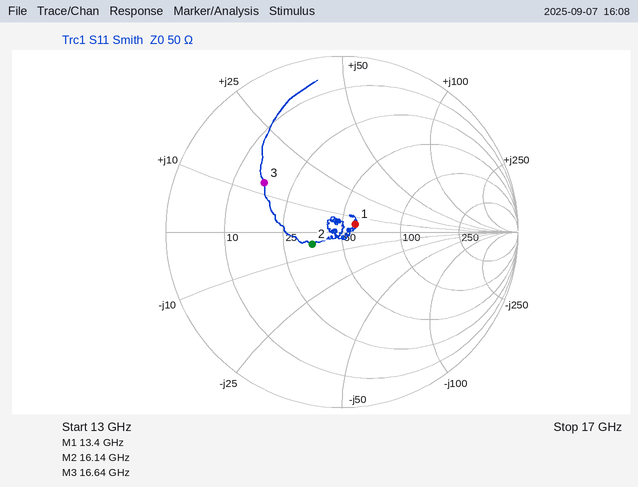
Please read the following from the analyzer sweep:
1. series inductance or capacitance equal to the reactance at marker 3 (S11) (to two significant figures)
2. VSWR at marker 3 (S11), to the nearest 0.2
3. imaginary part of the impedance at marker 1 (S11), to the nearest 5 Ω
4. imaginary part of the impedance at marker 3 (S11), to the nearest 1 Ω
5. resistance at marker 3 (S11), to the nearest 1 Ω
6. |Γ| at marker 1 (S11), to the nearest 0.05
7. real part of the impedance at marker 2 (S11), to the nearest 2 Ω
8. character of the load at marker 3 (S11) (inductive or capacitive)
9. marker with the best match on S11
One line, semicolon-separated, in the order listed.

120 pH; 3.2; +5 Ω; +13 Ω; 17 Ω; 0.10; 36 Ω; inductive; marker 1
